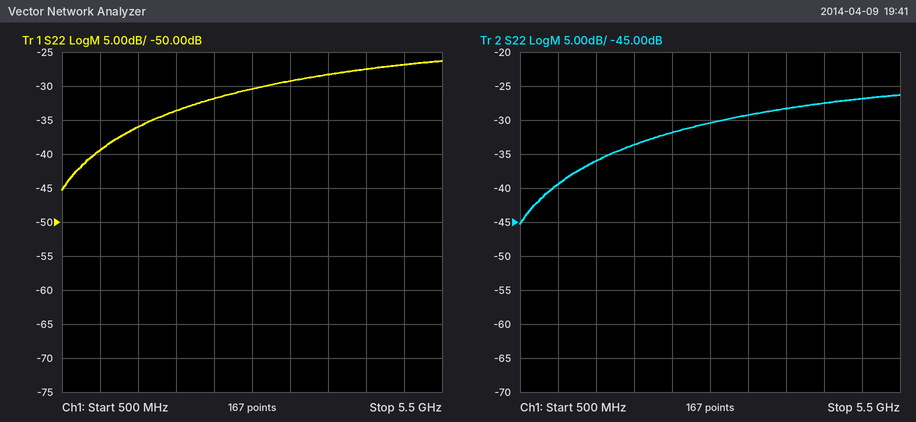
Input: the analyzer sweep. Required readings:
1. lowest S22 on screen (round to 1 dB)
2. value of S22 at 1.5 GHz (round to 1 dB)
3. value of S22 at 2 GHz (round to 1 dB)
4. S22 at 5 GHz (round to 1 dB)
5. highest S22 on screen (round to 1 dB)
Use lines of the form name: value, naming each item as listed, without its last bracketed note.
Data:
lowest S22 on screen: -45 dB
value of S22 at 1.5 GHz: -36 dB
value of S22 at 2 GHz: -34 dB
S22 at 5 GHz: -27 dB
highest S22 on screen: -26 dB
